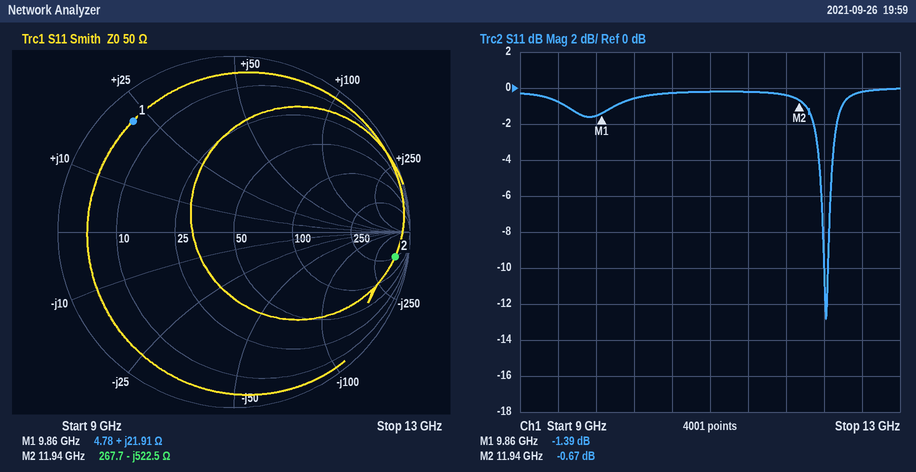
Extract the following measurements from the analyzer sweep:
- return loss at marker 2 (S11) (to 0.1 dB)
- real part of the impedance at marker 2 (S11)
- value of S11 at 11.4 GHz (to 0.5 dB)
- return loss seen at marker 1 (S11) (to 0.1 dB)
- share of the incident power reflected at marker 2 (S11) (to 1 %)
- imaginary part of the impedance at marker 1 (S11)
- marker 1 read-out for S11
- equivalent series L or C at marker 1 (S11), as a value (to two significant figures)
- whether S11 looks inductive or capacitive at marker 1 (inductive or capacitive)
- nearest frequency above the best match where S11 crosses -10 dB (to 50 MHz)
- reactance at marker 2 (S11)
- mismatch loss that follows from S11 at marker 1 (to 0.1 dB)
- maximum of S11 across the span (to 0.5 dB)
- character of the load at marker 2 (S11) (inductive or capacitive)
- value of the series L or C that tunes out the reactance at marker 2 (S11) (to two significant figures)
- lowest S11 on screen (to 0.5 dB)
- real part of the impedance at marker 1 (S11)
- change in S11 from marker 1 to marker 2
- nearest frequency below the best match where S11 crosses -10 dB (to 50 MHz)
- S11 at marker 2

0.7 dB
267.7 Ω
0.0 dB
1.4 dB
86 %
+21.91 Ω
-1.39 dB
350 pH
inductive
12.25 GHz
-522.5 Ω
5.6 dB
0.0 dB
capacitive
7.0 nH
-13.0 dB
4.78 Ω
0.72 dB
12.20 GHz
-0.67 dB
